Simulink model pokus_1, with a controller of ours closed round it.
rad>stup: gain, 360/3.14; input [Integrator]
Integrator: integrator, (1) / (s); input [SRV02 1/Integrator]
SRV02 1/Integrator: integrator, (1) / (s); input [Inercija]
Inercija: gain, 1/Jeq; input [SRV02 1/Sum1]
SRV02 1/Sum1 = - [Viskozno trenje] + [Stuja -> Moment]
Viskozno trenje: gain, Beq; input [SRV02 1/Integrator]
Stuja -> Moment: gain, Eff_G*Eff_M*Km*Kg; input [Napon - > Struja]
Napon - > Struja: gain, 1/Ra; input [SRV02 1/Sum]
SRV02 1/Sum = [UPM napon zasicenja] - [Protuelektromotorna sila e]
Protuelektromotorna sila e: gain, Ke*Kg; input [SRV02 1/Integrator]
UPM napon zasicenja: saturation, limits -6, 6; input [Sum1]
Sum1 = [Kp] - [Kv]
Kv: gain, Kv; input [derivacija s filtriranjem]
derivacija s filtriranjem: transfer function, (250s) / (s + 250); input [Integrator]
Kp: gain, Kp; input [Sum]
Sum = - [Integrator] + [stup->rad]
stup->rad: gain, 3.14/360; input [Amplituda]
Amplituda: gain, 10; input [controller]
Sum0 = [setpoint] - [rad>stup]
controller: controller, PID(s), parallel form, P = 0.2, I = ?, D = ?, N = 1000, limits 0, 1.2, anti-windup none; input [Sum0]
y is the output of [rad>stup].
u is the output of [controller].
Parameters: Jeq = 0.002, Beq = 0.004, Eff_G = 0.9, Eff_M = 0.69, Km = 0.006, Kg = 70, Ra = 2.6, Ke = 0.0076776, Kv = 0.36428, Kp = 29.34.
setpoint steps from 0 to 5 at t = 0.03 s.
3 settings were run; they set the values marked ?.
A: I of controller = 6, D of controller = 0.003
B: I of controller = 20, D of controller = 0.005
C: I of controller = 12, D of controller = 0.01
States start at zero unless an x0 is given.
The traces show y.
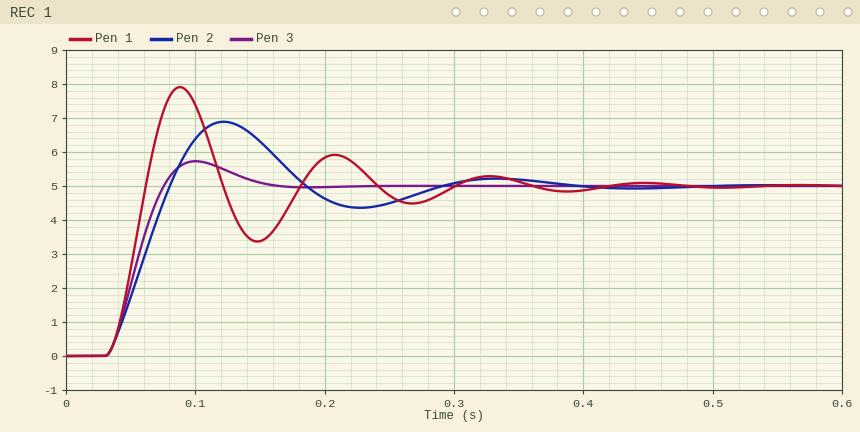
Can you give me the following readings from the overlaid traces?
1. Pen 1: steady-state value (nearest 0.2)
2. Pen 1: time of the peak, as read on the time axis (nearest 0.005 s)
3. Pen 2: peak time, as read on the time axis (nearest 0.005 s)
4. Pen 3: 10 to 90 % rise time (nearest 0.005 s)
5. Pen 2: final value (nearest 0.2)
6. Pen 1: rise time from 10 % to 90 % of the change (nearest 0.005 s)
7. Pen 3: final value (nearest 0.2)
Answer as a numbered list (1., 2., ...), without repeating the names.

1. 5.0
2. 0.090 s
3. 0.120 s
4. 0.030 s
5. 5.0
6. 0.020 s
7. 5.0
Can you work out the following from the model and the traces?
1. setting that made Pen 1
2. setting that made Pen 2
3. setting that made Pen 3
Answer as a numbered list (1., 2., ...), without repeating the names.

1. B
2. C
3. A
